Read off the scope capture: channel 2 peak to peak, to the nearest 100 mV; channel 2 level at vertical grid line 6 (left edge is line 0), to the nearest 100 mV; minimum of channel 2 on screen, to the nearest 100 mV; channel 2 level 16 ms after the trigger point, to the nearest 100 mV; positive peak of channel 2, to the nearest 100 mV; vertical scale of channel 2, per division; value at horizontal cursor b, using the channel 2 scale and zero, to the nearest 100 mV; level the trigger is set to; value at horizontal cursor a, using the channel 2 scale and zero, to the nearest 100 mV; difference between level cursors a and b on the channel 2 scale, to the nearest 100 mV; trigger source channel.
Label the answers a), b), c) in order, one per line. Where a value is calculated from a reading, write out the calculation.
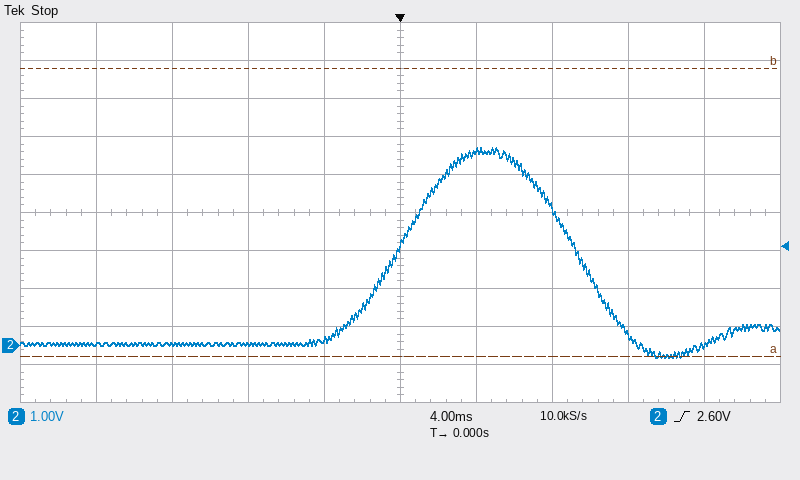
a) 5.2 V − (-300 mV) = 5.5 V
b) 5.1 V
c) -300 mV
d) 0.0 V
e) 5.2 V
f) 1 V
g) 7.3 V
h) 2.60 V
i) -300 mV
j) 7.6 V
k) channel 2
